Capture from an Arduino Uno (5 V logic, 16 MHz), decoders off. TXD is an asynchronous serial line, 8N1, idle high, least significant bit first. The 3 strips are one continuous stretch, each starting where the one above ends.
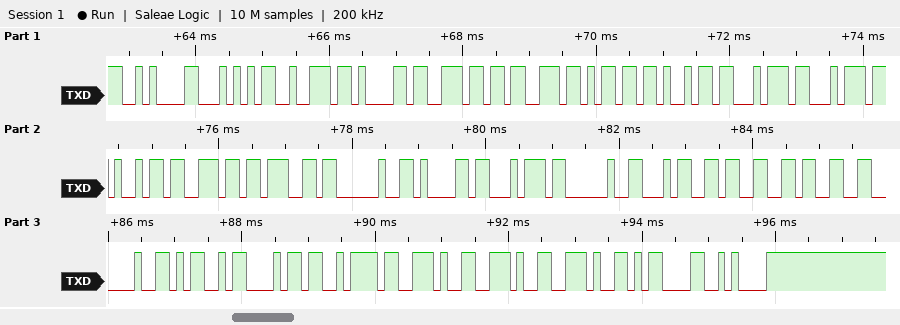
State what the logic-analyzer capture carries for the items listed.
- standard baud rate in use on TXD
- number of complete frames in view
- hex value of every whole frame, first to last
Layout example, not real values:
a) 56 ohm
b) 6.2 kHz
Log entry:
a) 9600 baud
b) 29
c) 0x0A 0x54 0x72 0x61 0x6E 0x73 0x6D 0x69 0x74 0x74 0x69 0x6E 0x67 0x20 0x61 0x74 0x20 0x34 0x33 0x33 0x20 0x4D 0x68 0x7A 0x2E 0x2E 0x2E 0x0D 0x0A
